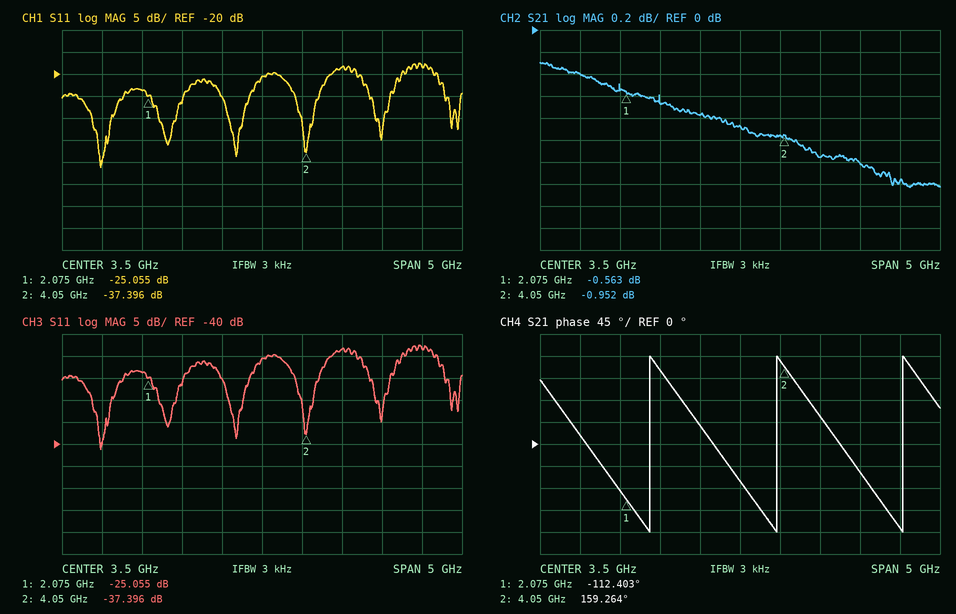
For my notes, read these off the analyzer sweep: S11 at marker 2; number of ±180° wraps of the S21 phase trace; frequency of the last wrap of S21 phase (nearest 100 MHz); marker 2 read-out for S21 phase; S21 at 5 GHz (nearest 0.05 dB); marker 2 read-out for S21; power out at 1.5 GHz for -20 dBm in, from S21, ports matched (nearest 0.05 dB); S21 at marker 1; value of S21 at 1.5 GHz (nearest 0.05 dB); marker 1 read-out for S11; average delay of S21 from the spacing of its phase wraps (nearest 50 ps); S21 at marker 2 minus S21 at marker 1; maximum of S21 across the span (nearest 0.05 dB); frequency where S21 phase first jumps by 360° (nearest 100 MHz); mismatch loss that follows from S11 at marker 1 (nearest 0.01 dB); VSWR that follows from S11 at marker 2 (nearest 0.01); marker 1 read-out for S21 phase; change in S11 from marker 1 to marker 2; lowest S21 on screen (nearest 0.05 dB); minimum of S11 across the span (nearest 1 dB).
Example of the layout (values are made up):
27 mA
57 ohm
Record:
-37.396 dB
3
5.5 GHz
159.264°
-1.20 dB
-0.952 dB
-20.40 dBm
-0.563 dB
-0.40 dB
-25.055 dB
650 ps
-0.389 dB
-0.30 dB
2.4 GHz
0.01 dB
1.03
-112.403°
-12.341 dB
-1.45 dB
-41 dB
